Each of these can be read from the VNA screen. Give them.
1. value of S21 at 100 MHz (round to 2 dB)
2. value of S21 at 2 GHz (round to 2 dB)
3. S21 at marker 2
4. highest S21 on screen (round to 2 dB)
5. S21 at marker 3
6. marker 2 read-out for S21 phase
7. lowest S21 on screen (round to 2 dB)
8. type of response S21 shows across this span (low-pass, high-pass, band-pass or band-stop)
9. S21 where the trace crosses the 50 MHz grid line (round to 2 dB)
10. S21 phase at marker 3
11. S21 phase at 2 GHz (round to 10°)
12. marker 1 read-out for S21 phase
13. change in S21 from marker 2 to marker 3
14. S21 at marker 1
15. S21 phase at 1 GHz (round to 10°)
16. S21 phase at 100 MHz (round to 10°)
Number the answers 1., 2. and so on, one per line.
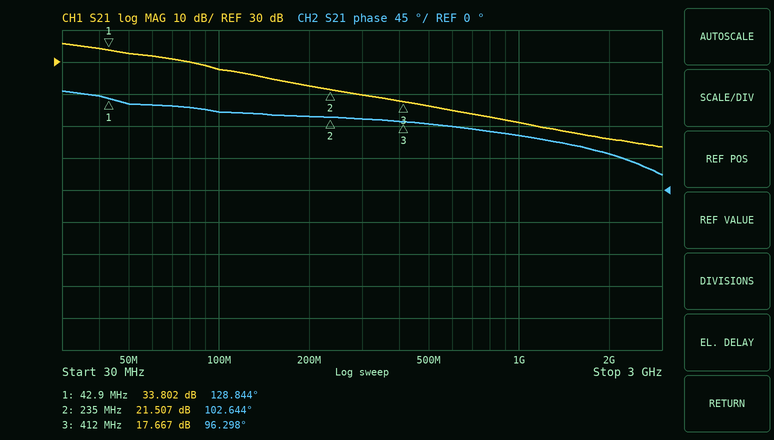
1. 28 dB
2. 6 dB
3. 21.507 dB
4. 36 dB
5. 17.667 dB
6. 102.644°
7. 4 dB
8. low-pass
9. 32 dB
10. 96.298°
11. 50°
12. 128.844°
13. -3.840 dB
14. 33.802 dB
15. 80°
16. 110°
